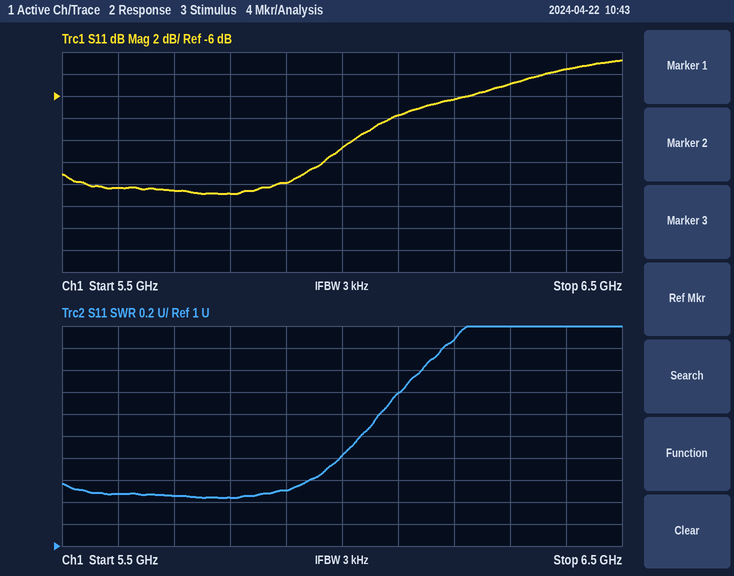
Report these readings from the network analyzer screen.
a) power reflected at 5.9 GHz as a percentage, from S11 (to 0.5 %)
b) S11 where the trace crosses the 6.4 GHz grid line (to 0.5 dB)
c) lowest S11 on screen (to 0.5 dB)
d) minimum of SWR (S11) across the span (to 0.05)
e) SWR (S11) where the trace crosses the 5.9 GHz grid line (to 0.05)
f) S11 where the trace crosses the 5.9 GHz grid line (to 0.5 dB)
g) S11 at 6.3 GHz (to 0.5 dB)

4.0 %
-3.5 dB
-15.0 dB
1.45
1.50
-14.0 dB
-5.0 dB
